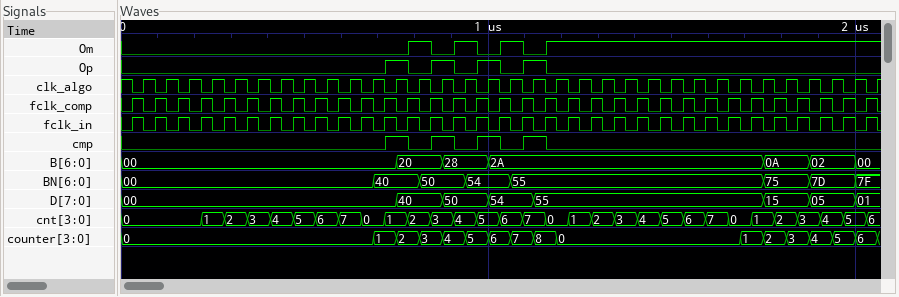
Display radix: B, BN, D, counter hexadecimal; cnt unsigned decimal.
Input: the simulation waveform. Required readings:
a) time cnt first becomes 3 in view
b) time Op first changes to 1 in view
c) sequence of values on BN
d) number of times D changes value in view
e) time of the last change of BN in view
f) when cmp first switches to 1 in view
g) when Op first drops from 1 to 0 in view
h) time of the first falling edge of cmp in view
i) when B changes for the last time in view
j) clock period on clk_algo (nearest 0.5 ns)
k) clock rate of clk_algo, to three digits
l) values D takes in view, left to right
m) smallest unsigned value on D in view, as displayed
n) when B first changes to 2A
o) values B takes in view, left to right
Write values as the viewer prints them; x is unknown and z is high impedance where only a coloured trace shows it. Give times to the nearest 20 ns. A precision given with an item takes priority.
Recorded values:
340 ns
720 ns
00, 40, 50, 54, 55, 75, 7D, 7F
7
2000 ns
720 ns
780 ns
780 ns
2000 ns
62.5 ns
16.0 MHz
00, 40, 50, 54, 55, 15, 05, 01
00
1000 ns
00, 20, 28, 2A, 0A, 02, 00
